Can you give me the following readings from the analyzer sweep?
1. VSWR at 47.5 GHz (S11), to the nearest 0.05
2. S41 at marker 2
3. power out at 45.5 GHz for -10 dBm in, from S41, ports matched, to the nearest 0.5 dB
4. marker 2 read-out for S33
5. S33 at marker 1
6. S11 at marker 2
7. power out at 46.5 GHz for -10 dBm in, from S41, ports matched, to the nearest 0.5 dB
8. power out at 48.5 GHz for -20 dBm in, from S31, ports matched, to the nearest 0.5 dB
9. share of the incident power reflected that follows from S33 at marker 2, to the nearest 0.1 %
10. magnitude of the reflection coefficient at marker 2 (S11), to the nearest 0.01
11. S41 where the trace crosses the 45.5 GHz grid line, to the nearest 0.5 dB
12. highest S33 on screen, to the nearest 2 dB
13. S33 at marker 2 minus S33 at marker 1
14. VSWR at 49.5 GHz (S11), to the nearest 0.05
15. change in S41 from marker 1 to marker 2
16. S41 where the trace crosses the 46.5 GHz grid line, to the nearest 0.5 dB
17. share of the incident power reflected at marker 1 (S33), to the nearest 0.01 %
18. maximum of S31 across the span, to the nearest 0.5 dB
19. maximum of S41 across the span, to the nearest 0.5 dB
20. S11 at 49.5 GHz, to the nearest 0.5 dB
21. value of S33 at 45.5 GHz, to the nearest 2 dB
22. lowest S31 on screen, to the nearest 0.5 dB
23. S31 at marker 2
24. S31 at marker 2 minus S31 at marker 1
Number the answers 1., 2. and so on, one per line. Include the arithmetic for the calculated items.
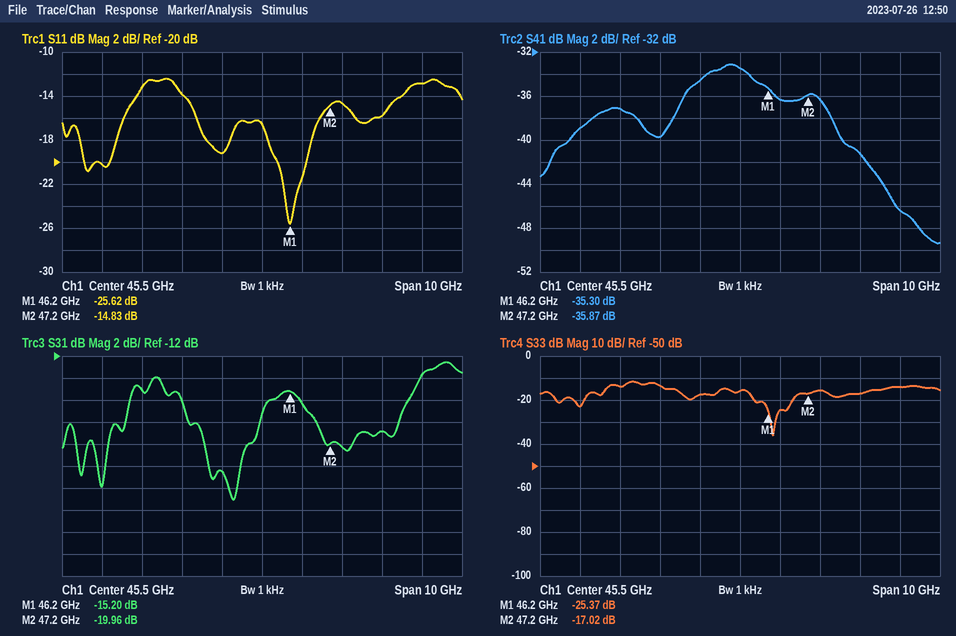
1. |Γ| = 10^(-14.5/20) = 0.1884; VSWR = (1 + 0.1884)/(1 − 0.1884) ≈ 1.46, so 1.45 to the nearest 0.05
2. -35.87 dB
3. -10 dBm + (-33.5 dB) = -43.5 dBm
4. -17.02 dB
5. -25.37 dB
6. -14.83 dB
7. -10 dBm + (-36.5 dB) = -46.5 dBm
8. -20 dBm + (-19.0 dB) = -39.0 dBm
9. 10^(-17.02/10) ≈ 2.0 %
10. 10^(-14.83/20) ≈ 0.18
11. -33.5 dB
12. -12 dB
13. -17.02 − (-25.37) = 8.35 dB
14. |Γ| = 10^(-13/20) = 0.2239; VSWR = (1 + 0.2239)/(1 − 0.2239) ≈ 1.58, so 1.60 to the nearest 0.05
15. -35.87 − (-35.3) = -0.57 dB
16. -36.5 dB
17. 10^(-25.37/10) ≈ 0.29 %
18. -12.5 dB
19. -33.0 dB
20. -13.0 dB
21. -16 dB
22. -25.0 dB
23. -19.96 dB
24. -19.96 − (-15.2) = -4.76 dB
